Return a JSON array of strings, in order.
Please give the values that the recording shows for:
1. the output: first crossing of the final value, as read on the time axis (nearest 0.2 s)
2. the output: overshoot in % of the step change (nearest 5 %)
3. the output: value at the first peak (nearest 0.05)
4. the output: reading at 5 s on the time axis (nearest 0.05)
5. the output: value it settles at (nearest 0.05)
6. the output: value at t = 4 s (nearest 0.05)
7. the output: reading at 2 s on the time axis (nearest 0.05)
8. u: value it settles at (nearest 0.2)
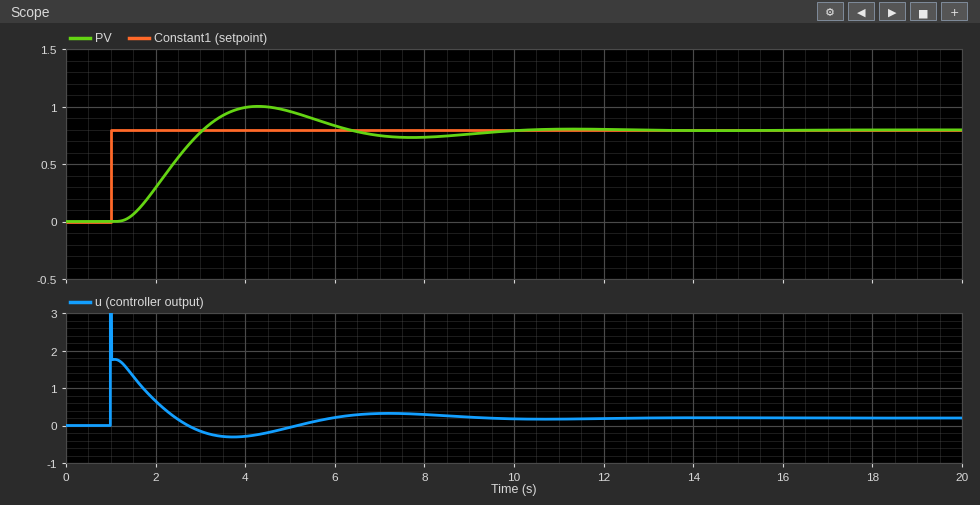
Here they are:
["3.0 s", "25 %", "1.00", "0.95", "0.80", "1.00", "0.30", "0.2"]
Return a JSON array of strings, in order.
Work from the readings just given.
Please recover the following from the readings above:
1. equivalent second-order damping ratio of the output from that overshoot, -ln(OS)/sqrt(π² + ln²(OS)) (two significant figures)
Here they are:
["0.40"]
